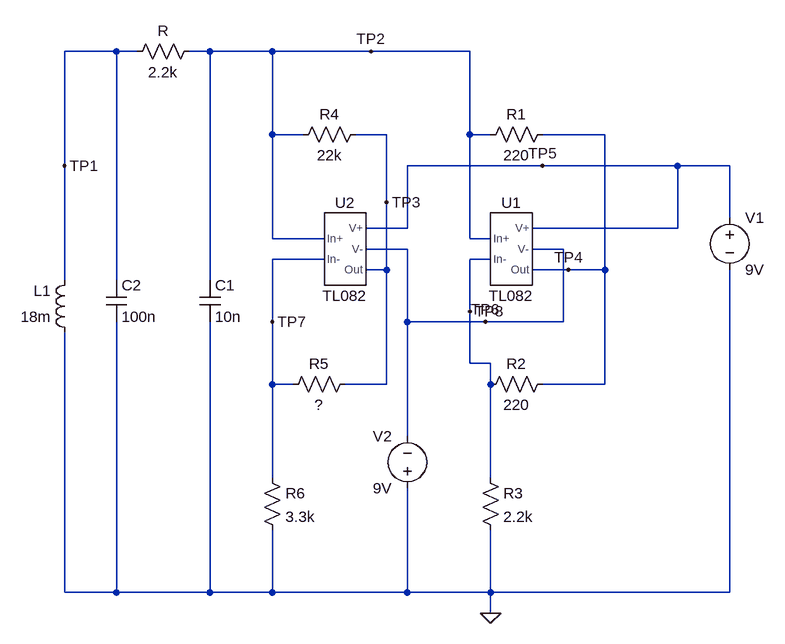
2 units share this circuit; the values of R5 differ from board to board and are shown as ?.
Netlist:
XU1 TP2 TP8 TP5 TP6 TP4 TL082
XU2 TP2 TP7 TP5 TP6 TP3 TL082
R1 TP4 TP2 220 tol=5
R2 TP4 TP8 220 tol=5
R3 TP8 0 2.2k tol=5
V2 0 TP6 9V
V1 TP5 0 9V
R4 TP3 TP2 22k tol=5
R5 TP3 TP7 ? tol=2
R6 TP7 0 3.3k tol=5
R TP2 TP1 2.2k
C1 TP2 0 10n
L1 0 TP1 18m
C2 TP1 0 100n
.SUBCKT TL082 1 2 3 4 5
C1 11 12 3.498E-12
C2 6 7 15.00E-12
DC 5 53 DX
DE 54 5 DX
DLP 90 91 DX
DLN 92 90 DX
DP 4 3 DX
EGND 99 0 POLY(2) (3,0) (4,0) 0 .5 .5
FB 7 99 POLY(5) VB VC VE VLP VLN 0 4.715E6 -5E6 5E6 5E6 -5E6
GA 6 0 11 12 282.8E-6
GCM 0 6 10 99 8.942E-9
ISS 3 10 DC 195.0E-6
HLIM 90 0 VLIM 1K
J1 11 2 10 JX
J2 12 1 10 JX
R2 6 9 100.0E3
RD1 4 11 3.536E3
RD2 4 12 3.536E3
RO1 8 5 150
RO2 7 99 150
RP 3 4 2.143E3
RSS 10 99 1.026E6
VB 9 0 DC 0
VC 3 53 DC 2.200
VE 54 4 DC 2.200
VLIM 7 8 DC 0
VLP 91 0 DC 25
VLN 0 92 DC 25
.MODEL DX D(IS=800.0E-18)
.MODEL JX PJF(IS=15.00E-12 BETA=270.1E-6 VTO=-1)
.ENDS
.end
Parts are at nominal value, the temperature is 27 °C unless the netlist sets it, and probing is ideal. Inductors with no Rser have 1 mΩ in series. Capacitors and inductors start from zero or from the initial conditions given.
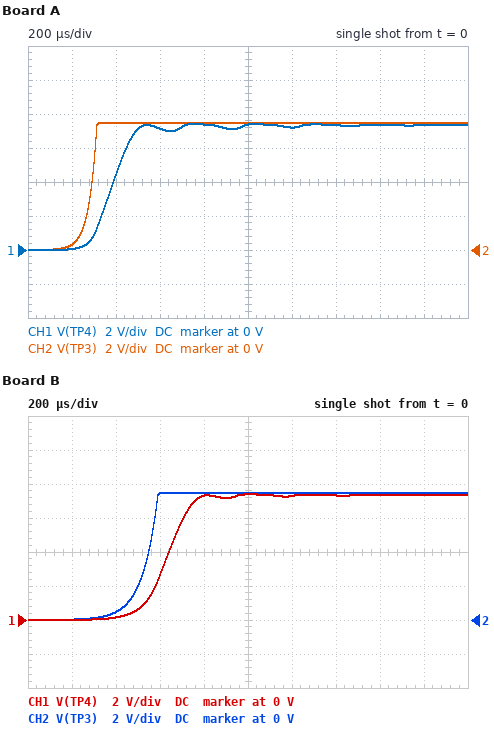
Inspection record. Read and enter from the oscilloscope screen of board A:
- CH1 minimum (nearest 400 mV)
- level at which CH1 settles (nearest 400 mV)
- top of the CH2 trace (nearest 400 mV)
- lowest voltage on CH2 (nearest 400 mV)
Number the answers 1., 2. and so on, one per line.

1. 0 V
2. 7.2 V
3. 7.6 V
4. 0 V
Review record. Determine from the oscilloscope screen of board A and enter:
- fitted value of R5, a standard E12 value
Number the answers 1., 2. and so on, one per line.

1. 18 kΩ
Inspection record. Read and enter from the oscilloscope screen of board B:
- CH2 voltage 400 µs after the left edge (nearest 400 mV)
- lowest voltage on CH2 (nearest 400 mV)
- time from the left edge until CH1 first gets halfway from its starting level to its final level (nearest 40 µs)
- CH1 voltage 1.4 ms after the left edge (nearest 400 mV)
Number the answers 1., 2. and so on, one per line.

1. 400 mV
2. 0 V
3. 640 µs
4. 7.2 V
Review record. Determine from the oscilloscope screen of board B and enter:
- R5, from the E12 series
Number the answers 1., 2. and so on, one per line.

1. 8.2 kΩ
